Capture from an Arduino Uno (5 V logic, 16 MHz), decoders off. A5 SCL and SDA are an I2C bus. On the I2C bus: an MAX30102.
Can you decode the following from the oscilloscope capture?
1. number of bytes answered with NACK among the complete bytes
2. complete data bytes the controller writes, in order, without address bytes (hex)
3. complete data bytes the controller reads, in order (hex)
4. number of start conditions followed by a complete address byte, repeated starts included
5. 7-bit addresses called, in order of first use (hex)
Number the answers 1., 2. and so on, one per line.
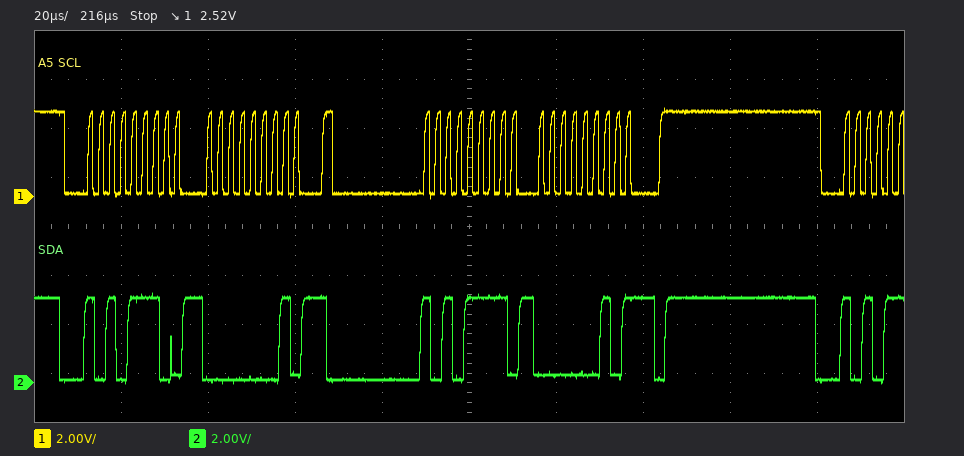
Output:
1. 1
2. 01
3. 02
4. 2
5. 0x57
